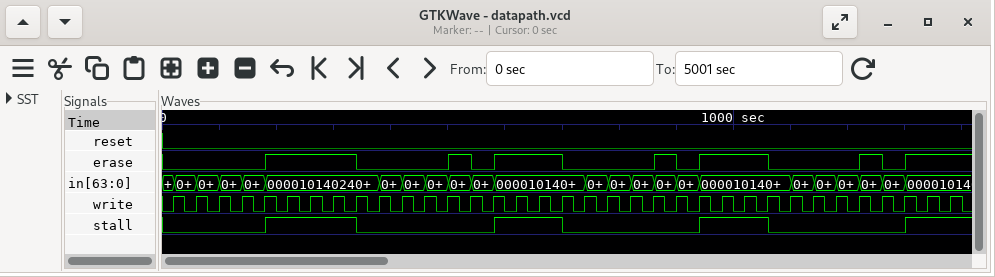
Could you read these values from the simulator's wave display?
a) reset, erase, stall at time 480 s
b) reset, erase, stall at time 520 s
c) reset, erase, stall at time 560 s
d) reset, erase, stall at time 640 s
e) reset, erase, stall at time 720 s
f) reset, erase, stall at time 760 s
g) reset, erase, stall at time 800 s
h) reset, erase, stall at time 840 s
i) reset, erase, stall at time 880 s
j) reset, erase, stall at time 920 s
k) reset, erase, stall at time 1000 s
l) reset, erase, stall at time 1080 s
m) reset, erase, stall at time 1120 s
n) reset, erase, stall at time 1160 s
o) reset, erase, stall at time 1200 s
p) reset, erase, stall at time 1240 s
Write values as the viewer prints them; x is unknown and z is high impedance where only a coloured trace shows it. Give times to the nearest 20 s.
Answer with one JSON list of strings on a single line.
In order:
["reset=0, erase=0, stall=0", "reset=0, erase=1, stall=0", "reset=0, erase=0, stall=0", "reset=0, erase=1, stall=1", "reset=0, erase=0, stall=0", "reset=0, erase=0, stall=0", "reset=0, erase=0, stall=0", "reset=0, erase=0, stall=0", "reset=0, erase=1, stall=0", "reset=0, erase=0, stall=0", "reset=0, erase=1, stall=1", "reset=0, erase=0, stall=0", "reset=0, erase=0, stall=0", "reset=0, erase=0, stall=0", "reset=0, erase=0, stall=0", "reset=0, erase=1, stall=0"]
